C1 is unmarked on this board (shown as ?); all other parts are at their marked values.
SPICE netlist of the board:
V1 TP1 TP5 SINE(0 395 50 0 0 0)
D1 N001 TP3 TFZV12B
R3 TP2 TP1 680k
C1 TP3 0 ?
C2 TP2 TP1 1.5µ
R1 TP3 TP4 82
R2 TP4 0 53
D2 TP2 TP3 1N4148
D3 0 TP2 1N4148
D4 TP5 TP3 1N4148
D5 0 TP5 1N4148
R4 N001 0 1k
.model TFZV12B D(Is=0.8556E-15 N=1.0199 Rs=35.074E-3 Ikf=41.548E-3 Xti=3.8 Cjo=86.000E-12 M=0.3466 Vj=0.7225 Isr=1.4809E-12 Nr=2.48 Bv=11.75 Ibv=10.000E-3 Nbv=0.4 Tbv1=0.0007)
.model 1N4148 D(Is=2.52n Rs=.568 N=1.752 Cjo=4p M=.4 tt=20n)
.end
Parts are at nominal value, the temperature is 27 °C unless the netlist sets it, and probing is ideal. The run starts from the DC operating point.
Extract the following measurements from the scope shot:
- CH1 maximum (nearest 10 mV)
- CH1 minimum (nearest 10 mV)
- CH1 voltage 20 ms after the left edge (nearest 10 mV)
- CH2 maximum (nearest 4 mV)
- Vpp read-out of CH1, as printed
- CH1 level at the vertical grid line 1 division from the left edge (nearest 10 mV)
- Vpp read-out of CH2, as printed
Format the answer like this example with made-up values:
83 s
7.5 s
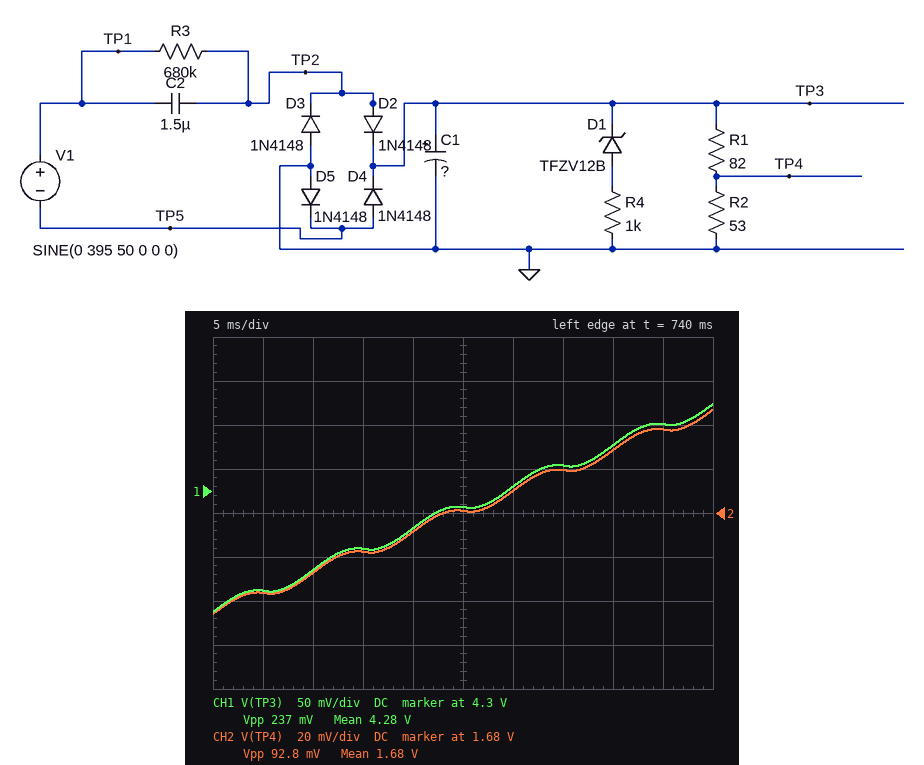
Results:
4.40 V
4.16 V
4.26 V
1.728 V
237 mV
4.19 V
92.8 mV
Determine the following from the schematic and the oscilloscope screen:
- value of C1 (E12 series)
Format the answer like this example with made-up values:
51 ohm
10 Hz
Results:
18 mF
